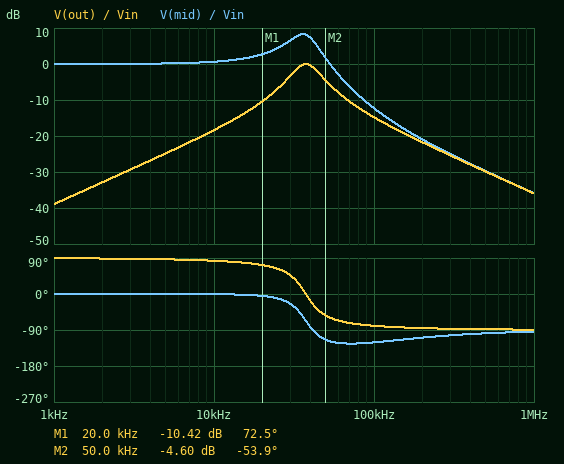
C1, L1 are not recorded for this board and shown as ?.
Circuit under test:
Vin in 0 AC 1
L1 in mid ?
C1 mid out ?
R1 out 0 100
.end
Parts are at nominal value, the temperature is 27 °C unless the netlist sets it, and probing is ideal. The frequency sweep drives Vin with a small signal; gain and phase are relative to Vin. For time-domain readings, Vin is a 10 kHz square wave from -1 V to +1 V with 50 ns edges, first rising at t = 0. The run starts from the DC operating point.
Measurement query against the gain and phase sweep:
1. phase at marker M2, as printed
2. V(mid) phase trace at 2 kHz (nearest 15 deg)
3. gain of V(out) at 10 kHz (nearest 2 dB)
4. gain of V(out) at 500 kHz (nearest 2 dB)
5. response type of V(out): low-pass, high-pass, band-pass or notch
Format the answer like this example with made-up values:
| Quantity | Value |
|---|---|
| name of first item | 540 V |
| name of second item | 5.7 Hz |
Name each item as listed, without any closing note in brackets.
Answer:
| Quantity | Value |
|---|---|
| phase at marker M2, as printed | -53.9 deg |
| V(mid) phase trace at 2 kHz | 0 deg |
| gain of V(out) at 10 kHz | -18 dB |
| gain of V(out) at 500 kHz | -30 dB |
| response type of V(out): low-pass, high-pass, band-pass or notch | band-pass |
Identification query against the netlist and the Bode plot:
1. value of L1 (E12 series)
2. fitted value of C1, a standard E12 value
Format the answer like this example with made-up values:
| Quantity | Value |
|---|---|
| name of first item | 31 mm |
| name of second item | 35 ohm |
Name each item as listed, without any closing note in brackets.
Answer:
| Quantity | Value |
|---|---|
| value of L1 | 1 mH |
| fitted value of C1, a standard E12 value | 18 nF |
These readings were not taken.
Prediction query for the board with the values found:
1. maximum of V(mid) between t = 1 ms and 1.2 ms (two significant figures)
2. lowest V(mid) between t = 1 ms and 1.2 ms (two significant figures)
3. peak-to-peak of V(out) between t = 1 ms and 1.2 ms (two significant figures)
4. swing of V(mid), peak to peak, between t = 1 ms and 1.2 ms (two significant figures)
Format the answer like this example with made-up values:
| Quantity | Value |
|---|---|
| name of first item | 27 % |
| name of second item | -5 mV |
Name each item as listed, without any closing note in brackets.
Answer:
| Quantity | Value |
|---|---|
| maximum of V(mid) between t = 1 ms and 1.2 ms | 2.1 V |
| lowest V(mid) between t = 1 ms and 1.2 ms | -2.1 V |
| peak-to-peak of V(out) between t = 1 ms and 1.2 ms | 1.2 V |
| swing of V(mid), peak to peak, between t = 1 ms and 1.2 ms | 4.2 V |
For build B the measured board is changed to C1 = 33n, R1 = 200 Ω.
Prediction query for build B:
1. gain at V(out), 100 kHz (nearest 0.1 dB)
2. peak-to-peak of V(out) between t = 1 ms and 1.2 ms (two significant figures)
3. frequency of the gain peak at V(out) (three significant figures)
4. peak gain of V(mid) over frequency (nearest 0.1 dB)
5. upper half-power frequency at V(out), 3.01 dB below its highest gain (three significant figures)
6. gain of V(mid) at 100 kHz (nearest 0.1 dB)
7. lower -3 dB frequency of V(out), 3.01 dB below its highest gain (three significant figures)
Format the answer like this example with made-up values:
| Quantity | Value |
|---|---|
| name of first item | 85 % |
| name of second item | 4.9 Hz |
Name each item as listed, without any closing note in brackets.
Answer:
| Quantity | Value |
|---|---|
| gain at V(out), 100 kHz | -9.7 dB |
| peak-to-peak of V(out) between t = 1 ms and 1.2 ms | 2.3 V |
| frequency of the gain peak at V(out) | 27.7 kHz |
| peak gain of V(mid) over frequency | 2.8 dB |
| upper half-power frequency at V(out), 3.01 dB below its highest gain | 47.9 kHz |
| gain of V(mid) at 100 kHz | -9.5 dB |
| lower -3 dB frequency of V(out), 3.01 dB below its highest gain | 16.0 kHz |
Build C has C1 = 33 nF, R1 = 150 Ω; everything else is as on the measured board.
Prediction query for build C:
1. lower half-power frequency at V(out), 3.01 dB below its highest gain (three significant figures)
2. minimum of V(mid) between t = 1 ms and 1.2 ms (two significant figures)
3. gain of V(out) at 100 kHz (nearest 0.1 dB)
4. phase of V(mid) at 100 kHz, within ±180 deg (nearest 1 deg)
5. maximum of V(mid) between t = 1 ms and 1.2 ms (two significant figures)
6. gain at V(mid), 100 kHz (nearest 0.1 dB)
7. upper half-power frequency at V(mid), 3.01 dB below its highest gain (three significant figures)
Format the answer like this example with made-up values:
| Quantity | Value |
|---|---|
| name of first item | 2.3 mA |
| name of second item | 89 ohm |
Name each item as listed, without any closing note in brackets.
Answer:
| Quantity | Value |
|---|---|
| lower half-power frequency at V(out), 3.01 dB below its highest gain | 18.2 kHz |
| minimum of V(mid) between t = 1 ms and 1.2 ms | -1.7 V |
| gain of V(out) at 100 kHz | -12.0 dB |
| phase of V(mid) at 100 kHz, within ±180 deg | -93 deg |
| maximum of V(mid) between t = 1 ms and 1.2 ms | 1.7 V |
| gain at V(mid), 100 kHz | -11.6 dB |
| upper half-power frequency at V(mid), 3.01 dB below its highest gain | 36.4 kHz |
